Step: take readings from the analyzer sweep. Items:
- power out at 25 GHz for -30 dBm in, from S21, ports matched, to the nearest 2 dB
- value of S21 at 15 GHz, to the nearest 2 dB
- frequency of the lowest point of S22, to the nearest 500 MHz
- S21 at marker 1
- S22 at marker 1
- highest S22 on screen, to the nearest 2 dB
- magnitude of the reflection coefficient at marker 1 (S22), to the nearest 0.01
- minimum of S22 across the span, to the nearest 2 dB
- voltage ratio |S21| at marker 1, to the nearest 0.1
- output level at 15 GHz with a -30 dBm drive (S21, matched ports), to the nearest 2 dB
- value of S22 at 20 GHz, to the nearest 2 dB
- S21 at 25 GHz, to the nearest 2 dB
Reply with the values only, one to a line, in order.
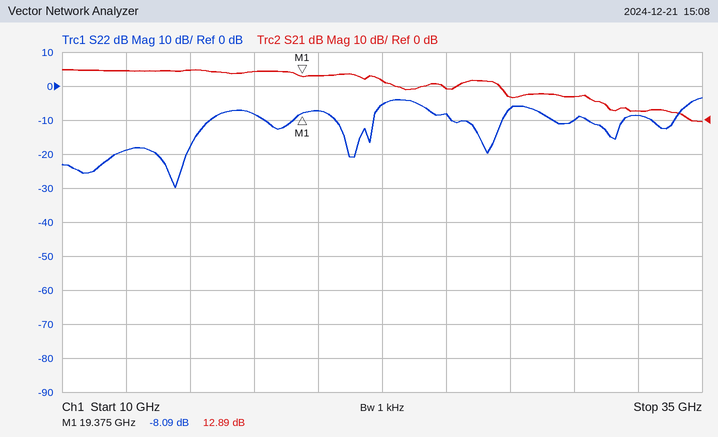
-20 dBm
14 dB
14.5 GHz
12.89 dB
-8.09 dB
-4 dB
0.39
-30 dB
4.4
-16 dBm
-8 dB
10 dB
